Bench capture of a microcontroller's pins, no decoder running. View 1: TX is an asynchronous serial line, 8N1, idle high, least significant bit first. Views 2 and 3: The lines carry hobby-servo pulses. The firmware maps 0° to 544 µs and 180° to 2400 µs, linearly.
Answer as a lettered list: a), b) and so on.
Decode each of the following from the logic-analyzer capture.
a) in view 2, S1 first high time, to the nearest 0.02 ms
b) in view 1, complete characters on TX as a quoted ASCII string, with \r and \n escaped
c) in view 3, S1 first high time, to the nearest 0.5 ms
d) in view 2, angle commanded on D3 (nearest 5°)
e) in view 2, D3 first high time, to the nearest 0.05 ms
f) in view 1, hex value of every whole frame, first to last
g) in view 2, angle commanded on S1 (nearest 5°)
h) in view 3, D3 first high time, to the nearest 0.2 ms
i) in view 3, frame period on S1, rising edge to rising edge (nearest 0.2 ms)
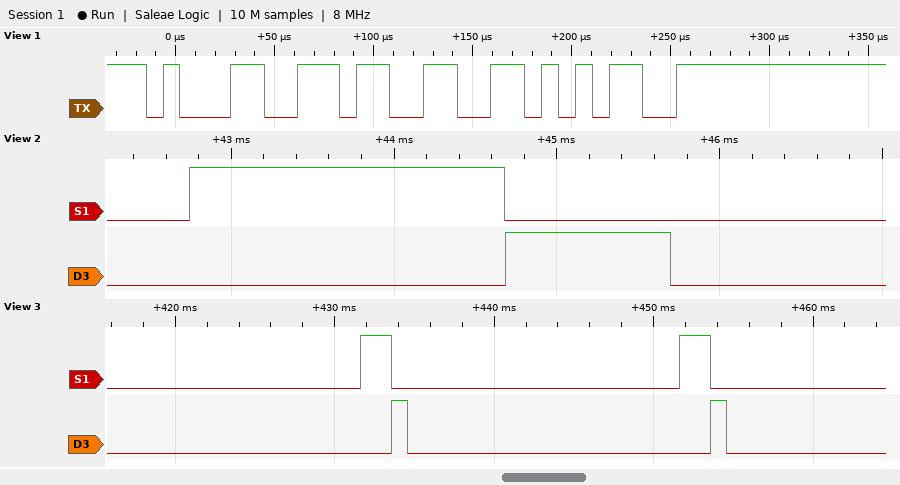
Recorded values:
a) 1.94 ms
b) "135"
c) 2.0 ms
d) 45°
e) 1.00 ms
f) 0x31 0x33 0x35
g) 135°
h) 1.0 ms
i) 20.0 ms
